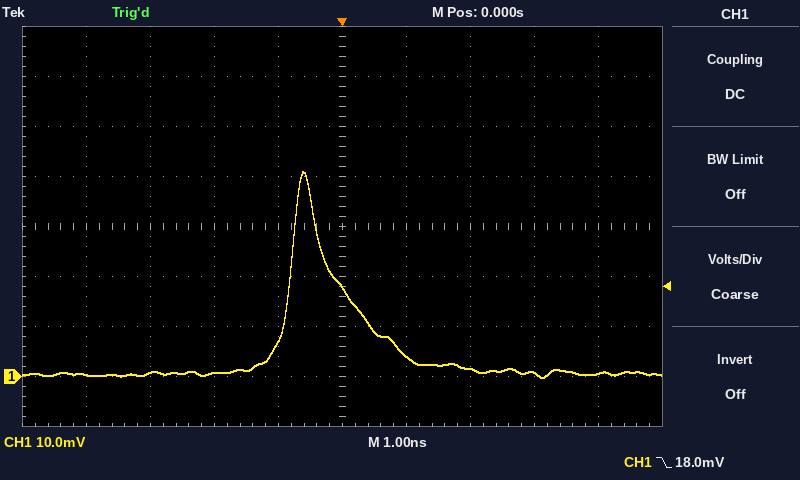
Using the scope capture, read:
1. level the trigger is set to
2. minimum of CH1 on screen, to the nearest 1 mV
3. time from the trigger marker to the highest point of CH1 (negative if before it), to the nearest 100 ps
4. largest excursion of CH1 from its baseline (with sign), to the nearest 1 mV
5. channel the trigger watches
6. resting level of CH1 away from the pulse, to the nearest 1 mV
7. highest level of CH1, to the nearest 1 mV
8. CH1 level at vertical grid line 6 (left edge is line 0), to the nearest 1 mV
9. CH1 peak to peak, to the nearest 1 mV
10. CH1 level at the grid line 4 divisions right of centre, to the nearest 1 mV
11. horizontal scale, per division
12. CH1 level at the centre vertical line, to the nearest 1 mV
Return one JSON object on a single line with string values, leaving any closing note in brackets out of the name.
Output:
{"level the trigger is set to": "18.0 mV", "minimum of CH1 on screen, to the nearest 1 mV": "0 mV", "time from the trigger marker to the highest point of CH1 (negative if before it), to the nearest 100 ps": "-600 ps", "largest excursion of CH1 from its baseline (with sign), to the nearest 1 mV": "+40 mV", "channel the trigger watches": "CH1", "resting level of CH1 away from the pulse, to the nearest 1 mV": "1 mV", "highest level of CH1, to the nearest 1 mV": "41 mV", "CH1 level at vertical grid line 6 (left edge is line 0), to the nearest 1 mV": "4 mV", "CH1 peak to peak, to the nearest 1 mV": "41 mV", "CH1 level at the grid line 4 divisions right of centre, to the nearest 1 mV": "1 mV", "horizontal scale, per division": "1 ns", "CH1 level at the centre vertical line, to the nearest 1 mV": "18 mV"}
